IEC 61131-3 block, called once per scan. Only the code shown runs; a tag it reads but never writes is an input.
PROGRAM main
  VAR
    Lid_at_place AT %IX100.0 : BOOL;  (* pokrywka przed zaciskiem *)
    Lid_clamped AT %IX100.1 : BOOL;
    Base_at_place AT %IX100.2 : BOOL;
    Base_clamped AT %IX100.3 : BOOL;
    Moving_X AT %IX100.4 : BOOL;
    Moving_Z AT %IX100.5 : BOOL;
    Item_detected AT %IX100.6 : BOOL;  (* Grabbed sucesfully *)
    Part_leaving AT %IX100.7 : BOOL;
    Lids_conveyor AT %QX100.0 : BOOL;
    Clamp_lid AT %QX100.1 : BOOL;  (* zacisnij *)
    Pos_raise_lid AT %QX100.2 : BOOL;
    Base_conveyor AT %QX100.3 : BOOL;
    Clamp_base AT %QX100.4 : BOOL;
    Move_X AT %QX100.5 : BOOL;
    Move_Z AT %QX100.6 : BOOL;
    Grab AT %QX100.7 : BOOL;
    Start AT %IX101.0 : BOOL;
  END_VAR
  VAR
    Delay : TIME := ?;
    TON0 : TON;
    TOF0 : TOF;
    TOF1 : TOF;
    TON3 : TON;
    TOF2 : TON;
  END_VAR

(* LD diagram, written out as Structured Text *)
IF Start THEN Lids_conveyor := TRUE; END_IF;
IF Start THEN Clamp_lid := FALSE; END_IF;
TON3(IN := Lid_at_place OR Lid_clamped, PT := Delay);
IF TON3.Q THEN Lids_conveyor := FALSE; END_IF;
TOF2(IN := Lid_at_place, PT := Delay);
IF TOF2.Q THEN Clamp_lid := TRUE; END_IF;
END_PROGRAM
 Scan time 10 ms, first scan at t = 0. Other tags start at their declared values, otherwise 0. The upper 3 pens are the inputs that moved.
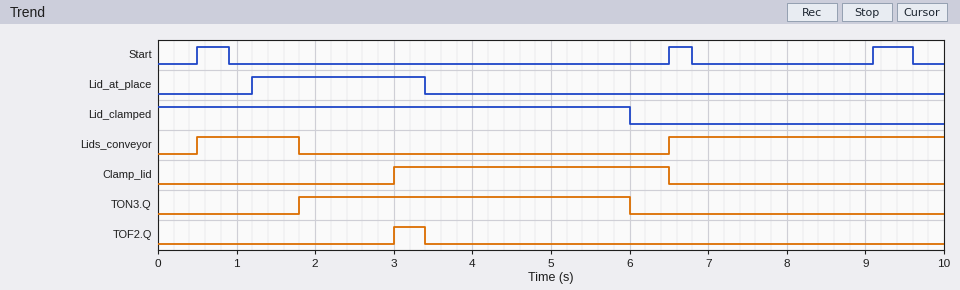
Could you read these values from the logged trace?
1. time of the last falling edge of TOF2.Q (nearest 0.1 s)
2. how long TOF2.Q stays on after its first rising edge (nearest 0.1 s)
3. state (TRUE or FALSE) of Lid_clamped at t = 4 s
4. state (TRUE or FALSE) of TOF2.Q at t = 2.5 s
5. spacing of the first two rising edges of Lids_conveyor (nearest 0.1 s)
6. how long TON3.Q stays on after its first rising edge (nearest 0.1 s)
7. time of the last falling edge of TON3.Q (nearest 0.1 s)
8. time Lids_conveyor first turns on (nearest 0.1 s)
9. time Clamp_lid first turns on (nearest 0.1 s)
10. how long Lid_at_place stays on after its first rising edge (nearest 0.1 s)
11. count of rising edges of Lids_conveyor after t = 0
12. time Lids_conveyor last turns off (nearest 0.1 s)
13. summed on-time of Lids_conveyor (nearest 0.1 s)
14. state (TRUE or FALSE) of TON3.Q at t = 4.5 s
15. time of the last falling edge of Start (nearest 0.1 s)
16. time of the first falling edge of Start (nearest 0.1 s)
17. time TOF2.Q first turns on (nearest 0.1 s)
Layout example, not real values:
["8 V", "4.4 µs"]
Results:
["3.4 s", "0.4 s", "TRUE", "FALSE", "6.0 s", "4.2 s", "6.0 s", "0.5 s", "3.0 s", "2.2 s", "2", "1.8 s", "4.8 s", "TRUE", "9.6 s", "0.9 s", "3.0 s"]
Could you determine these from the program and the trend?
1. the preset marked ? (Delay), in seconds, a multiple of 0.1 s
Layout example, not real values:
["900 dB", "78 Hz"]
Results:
["1.8 s"]
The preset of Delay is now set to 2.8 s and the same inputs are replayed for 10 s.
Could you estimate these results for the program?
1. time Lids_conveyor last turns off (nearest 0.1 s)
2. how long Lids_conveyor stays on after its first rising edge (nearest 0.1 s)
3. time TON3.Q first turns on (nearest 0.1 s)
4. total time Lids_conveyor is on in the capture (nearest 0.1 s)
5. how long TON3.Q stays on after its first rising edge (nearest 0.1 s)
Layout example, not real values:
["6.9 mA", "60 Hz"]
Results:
["2.8 s", "2.3 s", "2.8 s", "5.8 s", "3.2 s"]
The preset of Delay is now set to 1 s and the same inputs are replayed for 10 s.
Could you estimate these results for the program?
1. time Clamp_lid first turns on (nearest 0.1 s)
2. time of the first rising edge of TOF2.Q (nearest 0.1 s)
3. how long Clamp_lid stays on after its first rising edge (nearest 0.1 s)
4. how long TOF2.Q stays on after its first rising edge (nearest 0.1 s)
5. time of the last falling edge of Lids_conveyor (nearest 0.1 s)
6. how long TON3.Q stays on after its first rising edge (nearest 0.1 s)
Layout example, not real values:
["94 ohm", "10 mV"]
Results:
["2.2 s", "2.2 s", "4.3 s", "1.2 s", "1.0 s", "5.0 s"]
